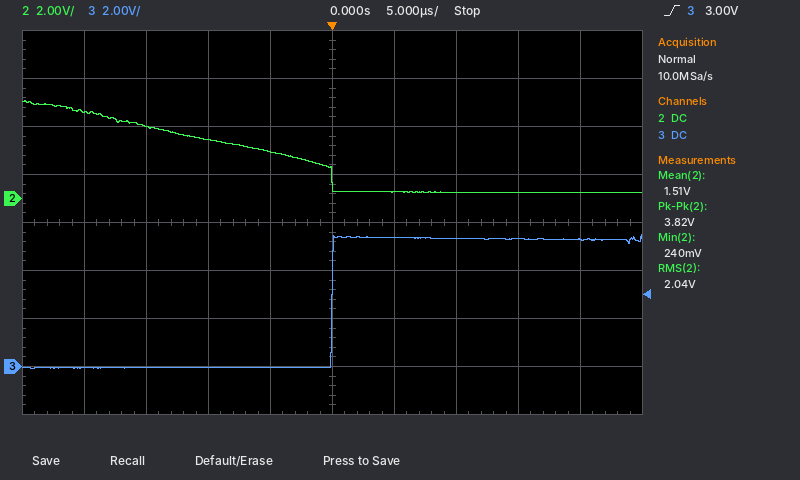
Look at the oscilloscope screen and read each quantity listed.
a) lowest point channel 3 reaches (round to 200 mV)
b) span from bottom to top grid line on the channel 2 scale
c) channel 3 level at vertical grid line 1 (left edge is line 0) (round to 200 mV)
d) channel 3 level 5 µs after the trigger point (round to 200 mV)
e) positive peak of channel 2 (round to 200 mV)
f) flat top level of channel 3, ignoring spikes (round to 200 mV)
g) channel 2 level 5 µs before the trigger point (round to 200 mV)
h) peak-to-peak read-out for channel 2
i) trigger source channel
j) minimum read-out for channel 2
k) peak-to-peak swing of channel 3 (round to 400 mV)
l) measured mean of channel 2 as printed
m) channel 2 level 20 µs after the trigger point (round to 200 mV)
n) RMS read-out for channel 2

0.0 V
16 V
0.0 V
5.4 V
4.0 V
5.4 V
2.0 V
3.82 V
channel 3
240 mV
5.6 V
1.51 V
200 mV
2.04 V
